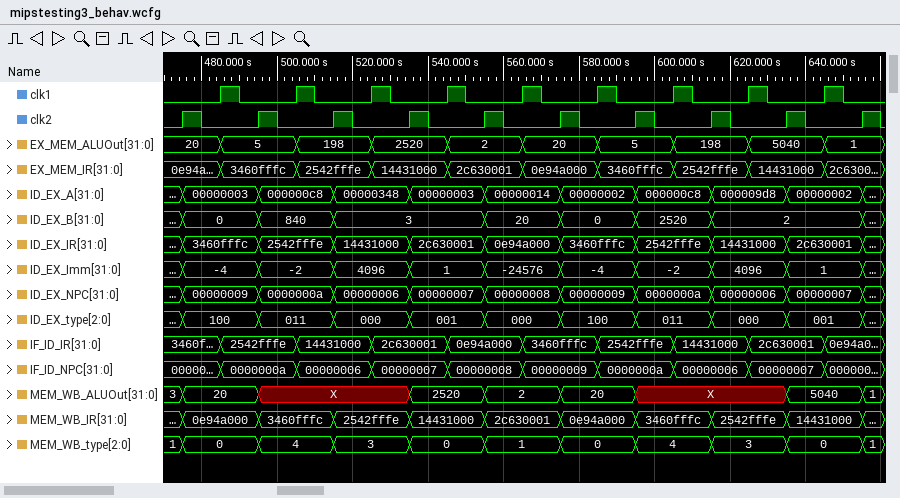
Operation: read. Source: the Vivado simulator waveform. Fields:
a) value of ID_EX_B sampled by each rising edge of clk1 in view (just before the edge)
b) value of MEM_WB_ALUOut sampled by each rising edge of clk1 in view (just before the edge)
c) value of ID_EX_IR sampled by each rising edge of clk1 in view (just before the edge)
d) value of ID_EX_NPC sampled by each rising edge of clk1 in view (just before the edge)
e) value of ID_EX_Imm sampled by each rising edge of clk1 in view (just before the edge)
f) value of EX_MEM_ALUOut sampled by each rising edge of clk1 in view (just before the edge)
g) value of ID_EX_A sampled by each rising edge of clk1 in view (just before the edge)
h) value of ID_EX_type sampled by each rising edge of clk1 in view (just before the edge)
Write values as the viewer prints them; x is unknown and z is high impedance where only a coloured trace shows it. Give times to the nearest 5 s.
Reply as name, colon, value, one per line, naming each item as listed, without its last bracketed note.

value of ID_EX_B sampled by each rising edge of clk1 in view: 0, 840, 3, 3, 20, 0, 2520, 2, 2
value of MEM_WB_ALUOut sampled by each rising edge of clk1 in view: 20, X, X, 2520, 2, 20, X, X, 5040
value of ID_EX_IR sampled by each rising edge of clk1 in view: 3460fffc, 2542fffe, 14431000, 2c630001, 0e94a000, 3460fffc, 2542fffe, 14431000, 2c630001
value of ID_EX_NPC sampled by each rising edge of clk1 in view: 00000009, 0000000a, 00000006, 00000007, 00000008, 00000009, 0000000a, 00000006, 00000007
value of ID_EX_Imm sampled by each rising edge of clk1 in view: -4, -2, 4096, 1, -24576, -4, -2, 4096, 1
value of EX_MEM_ALUOut sampled by each rising edge of clk1 in view: 20, 5, 198, 2520, 2, 20, 5, 198, 5040
value of ID_EX_A sampled by each rising edge of clk1 in view: 00000003, 000000c8, 00000348, 00000003, 00000014, 00000002, 000000c8, 000009d8, 00000002
value of ID_EX_type sampled by each rising edge of clk1 in view: 100, 011, 000, 001, 000, 100, 011, 000, 001
